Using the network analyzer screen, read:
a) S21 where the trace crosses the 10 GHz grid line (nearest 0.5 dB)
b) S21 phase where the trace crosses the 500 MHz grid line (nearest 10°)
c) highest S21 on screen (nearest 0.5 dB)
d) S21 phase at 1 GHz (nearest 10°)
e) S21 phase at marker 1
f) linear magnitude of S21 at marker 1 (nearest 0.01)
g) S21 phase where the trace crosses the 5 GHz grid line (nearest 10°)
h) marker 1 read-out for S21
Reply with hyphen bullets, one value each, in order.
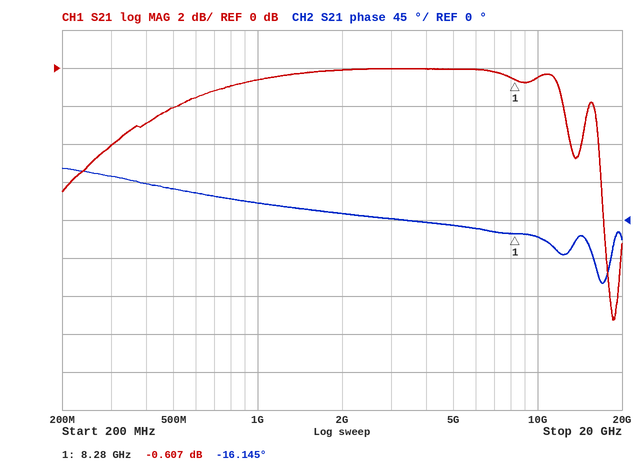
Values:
- -0.5 dB
- 40°
- 0.0 dB
- 20°
- -16.145°
- 0.93
- -10°
- -0.607 dB
